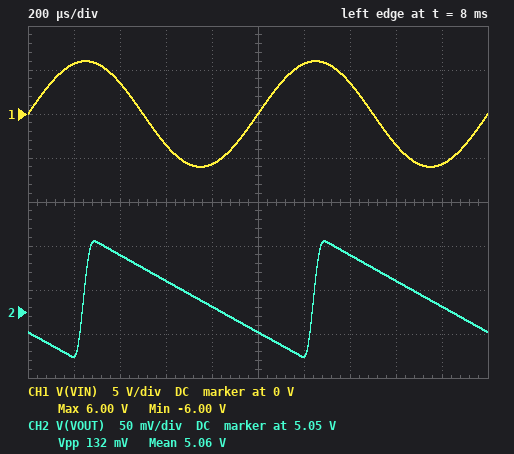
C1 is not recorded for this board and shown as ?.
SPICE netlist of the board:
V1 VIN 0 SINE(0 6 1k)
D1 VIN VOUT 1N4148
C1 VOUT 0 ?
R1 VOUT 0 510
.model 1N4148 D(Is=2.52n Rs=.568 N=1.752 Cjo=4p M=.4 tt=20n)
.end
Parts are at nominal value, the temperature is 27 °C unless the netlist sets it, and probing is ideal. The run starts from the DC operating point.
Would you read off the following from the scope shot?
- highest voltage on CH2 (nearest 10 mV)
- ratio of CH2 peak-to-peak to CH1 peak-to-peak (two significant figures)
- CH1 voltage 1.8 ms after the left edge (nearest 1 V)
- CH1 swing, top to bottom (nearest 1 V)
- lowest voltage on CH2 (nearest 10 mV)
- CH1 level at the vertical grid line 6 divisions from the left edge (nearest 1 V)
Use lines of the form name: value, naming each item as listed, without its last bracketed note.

highest voltage on CH2: 5.13 V
ratio of CH2 peak-to-peak to CH1 peak-to-peak: 0.011
CH1 voltage 1.8 ms after the left edge: -6 V
CH1 swing, top to bottom: 12 V
lowest voltage on CH2: 5.00 V
CH1 level at the vertical grid line 6 divisions from the left edge: 6 V
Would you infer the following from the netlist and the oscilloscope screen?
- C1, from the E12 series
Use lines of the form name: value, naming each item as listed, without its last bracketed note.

C1, from the E12 series: 68 µF
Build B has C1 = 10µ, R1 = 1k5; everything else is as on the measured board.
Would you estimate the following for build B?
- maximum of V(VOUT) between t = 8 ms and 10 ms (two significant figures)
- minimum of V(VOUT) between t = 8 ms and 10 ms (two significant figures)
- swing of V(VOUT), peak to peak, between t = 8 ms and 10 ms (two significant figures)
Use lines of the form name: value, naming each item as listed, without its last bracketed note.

maximum of V(VOUT) between t = 8 ms and 10 ms: 5.3 V
minimum of V(VOUT) between t = 8 ms and 10 ms: 5.0 V
swing of V(VOUT), peak to peak, between t = 8 ms and 10 ms: 310 mV
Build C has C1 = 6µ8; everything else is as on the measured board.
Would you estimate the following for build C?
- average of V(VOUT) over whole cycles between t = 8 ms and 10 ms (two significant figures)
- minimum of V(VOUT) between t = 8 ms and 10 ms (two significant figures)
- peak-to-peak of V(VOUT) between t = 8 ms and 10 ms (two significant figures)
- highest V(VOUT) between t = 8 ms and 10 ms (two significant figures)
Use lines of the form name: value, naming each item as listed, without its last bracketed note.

average of V(VOUT) over whole cycles between t = 8 ms and 10 ms: 4.7 V
minimum of V(VOUT) between t = 8 ms and 10 ms: 4.1 V
peak-to-peak of V(VOUT) between t = 8 ms and 10 ms: 1.2 V
highest V(VOUT) between t = 8 ms and 10 ms: 5.3 V
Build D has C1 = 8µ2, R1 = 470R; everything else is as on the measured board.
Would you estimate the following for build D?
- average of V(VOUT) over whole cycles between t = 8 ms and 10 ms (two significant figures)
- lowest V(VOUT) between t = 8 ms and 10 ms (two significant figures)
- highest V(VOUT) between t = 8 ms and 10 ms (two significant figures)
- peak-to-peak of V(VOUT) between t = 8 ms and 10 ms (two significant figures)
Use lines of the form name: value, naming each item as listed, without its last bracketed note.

average of V(VOUT) over whole cycles between t = 8 ms and 10 ms: 4.7 V
lowest V(VOUT) between t = 8 ms and 10 ms: 4.2 V
highest V(VOUT) between t = 8 ms and 10 ms: 5.3 V
peak-to-peak of V(VOUT) between t = 8 ms and 10 ms: 1.1 V
